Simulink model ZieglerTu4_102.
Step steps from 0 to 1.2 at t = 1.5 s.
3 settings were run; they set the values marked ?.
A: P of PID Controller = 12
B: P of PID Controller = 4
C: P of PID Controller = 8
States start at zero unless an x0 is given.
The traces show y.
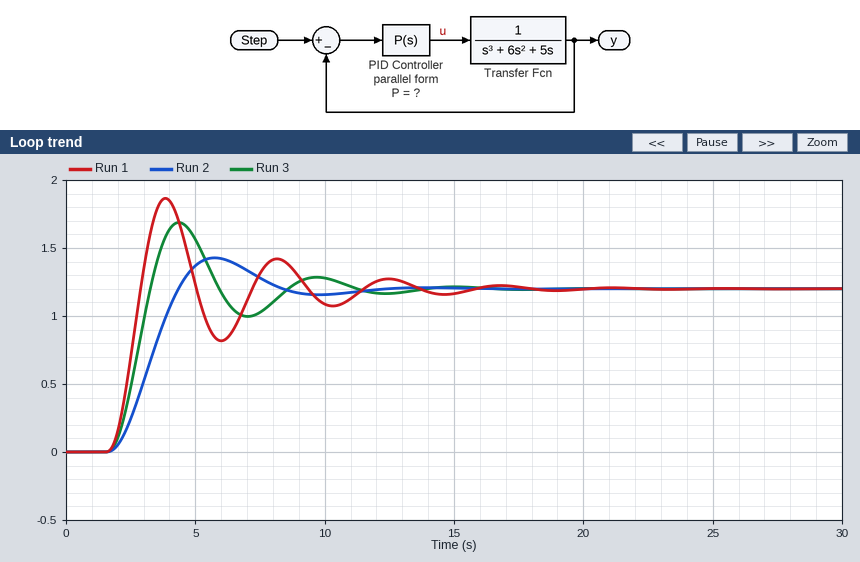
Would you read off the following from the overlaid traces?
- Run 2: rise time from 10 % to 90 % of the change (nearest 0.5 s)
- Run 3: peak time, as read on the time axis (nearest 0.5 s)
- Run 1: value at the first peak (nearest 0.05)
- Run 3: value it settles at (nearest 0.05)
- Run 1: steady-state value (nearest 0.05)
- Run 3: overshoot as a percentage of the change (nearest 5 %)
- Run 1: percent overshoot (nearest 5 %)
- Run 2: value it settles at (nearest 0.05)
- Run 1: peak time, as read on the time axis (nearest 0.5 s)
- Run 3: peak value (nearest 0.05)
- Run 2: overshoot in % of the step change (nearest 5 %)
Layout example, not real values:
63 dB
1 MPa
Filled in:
2.0 s
4.5 s
1.85
1.20
1.20
40 %
55 %
1.20
4.0 s
1.70
20 %
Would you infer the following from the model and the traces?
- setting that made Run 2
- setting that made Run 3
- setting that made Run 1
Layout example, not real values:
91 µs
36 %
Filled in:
B
C
A
